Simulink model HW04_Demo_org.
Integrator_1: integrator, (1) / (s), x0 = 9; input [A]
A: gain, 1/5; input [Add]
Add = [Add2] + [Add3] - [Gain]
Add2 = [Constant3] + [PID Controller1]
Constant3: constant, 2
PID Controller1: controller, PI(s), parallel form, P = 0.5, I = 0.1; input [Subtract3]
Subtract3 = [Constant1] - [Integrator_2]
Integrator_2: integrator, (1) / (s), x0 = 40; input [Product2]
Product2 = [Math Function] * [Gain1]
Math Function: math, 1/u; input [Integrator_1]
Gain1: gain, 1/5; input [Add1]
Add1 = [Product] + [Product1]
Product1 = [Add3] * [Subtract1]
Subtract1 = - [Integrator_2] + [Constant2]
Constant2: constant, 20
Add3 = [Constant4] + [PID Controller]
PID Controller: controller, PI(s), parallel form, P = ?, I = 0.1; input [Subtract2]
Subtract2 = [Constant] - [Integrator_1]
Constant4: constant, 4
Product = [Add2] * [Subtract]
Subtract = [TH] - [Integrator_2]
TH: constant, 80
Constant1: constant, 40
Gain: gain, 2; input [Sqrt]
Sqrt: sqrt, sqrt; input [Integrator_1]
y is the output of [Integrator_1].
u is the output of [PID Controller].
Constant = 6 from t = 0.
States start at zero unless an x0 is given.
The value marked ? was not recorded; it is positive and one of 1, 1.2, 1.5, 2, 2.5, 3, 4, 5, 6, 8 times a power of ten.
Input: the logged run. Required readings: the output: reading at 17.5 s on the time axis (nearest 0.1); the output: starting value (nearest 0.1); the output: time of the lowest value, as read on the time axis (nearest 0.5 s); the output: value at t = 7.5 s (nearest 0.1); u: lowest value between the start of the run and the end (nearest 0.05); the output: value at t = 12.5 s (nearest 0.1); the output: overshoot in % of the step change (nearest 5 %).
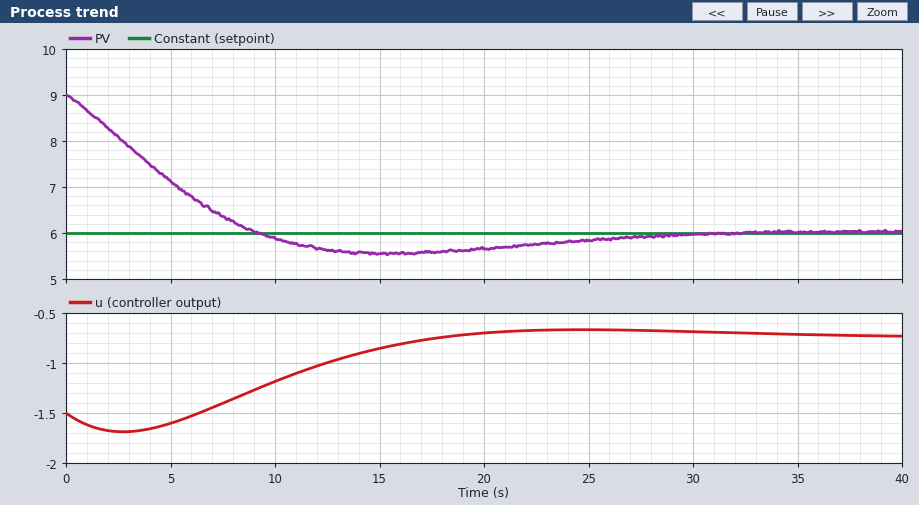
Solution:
5.6
9.0
15.5 s
6.4
-1.70
5.6
15 %
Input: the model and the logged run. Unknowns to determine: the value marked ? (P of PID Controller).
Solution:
0.5
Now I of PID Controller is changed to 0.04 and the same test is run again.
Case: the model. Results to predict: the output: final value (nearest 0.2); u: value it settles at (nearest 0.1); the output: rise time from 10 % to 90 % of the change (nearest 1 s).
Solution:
6.0
-0.7
12 s
